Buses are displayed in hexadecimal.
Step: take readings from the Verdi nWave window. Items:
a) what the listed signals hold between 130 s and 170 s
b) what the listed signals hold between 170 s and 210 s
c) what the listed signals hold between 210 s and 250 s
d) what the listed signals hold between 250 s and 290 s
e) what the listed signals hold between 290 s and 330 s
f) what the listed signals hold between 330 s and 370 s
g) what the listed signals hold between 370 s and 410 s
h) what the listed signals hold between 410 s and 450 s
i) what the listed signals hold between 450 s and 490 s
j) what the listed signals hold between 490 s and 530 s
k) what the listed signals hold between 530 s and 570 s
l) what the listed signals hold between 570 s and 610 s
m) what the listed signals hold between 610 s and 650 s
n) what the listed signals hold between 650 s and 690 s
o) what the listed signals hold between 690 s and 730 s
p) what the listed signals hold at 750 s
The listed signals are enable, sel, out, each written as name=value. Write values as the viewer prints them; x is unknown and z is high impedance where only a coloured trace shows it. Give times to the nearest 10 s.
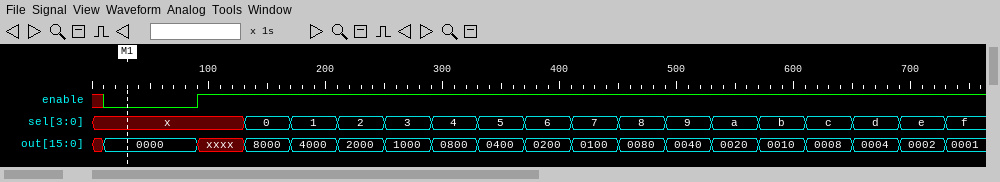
enable=1, sel=0, out=8000
enable=1, sel=1, out=4000
enable=1, sel=2, out=2000
enable=1, sel=3, out=1000
enable=1, sel=4, out=0800
enable=1, sel=5, out=0400
enable=1, sel=6, out=0200
enable=1, sel=7, out=0100
enable=1, sel=8, out=0080
enable=1, sel=9, out=0040
enable=1, sel=a, out=0020
enable=1, sel=b, out=0010
enable=1, sel=c, out=0008
enable=1, sel=d, out=0004
enable=1, sel=e, out=0002
enable=1, sel=f, out=0001
